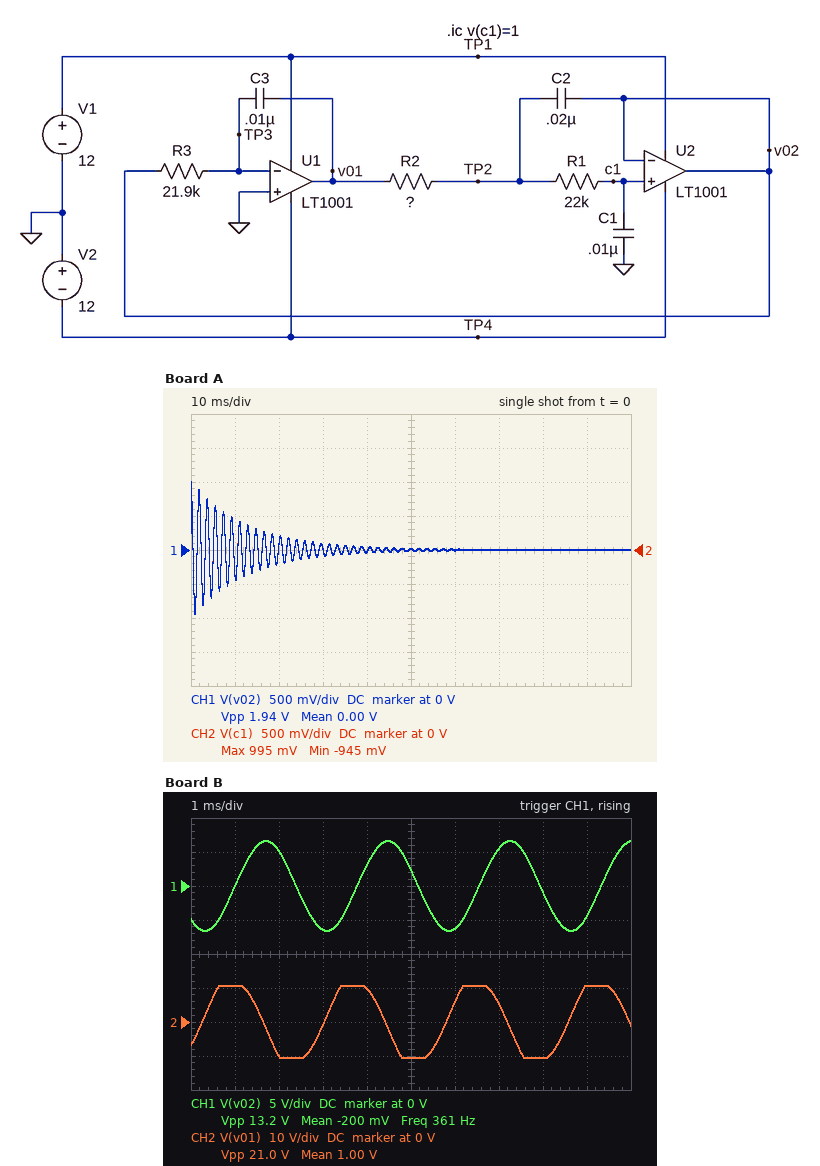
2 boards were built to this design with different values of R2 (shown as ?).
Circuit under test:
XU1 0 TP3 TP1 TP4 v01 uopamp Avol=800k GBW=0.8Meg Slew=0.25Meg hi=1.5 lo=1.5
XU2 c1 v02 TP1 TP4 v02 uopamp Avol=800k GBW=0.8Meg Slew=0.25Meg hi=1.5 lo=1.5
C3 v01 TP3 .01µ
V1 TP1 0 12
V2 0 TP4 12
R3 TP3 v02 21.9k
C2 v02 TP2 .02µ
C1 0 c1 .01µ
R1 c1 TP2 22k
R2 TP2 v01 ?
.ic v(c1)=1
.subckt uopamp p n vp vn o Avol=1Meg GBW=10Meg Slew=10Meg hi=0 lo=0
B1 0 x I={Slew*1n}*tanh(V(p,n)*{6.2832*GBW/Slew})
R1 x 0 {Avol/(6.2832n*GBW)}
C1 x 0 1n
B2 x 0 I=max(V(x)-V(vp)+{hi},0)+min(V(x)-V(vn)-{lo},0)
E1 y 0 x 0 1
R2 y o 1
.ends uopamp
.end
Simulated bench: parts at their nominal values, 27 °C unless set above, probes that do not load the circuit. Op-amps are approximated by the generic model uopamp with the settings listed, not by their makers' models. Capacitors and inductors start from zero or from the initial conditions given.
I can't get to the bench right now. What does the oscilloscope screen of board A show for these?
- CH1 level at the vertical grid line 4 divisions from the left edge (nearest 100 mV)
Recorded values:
0 V
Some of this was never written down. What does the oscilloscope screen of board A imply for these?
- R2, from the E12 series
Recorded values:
18 kΩ
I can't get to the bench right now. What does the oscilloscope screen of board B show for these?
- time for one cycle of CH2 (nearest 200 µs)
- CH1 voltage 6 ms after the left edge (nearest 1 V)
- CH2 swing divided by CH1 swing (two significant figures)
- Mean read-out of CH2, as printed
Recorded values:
2.8 ms
-6 V
1.6
1.00 V
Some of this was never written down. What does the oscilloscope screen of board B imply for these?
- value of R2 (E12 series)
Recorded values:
56 kΩ
